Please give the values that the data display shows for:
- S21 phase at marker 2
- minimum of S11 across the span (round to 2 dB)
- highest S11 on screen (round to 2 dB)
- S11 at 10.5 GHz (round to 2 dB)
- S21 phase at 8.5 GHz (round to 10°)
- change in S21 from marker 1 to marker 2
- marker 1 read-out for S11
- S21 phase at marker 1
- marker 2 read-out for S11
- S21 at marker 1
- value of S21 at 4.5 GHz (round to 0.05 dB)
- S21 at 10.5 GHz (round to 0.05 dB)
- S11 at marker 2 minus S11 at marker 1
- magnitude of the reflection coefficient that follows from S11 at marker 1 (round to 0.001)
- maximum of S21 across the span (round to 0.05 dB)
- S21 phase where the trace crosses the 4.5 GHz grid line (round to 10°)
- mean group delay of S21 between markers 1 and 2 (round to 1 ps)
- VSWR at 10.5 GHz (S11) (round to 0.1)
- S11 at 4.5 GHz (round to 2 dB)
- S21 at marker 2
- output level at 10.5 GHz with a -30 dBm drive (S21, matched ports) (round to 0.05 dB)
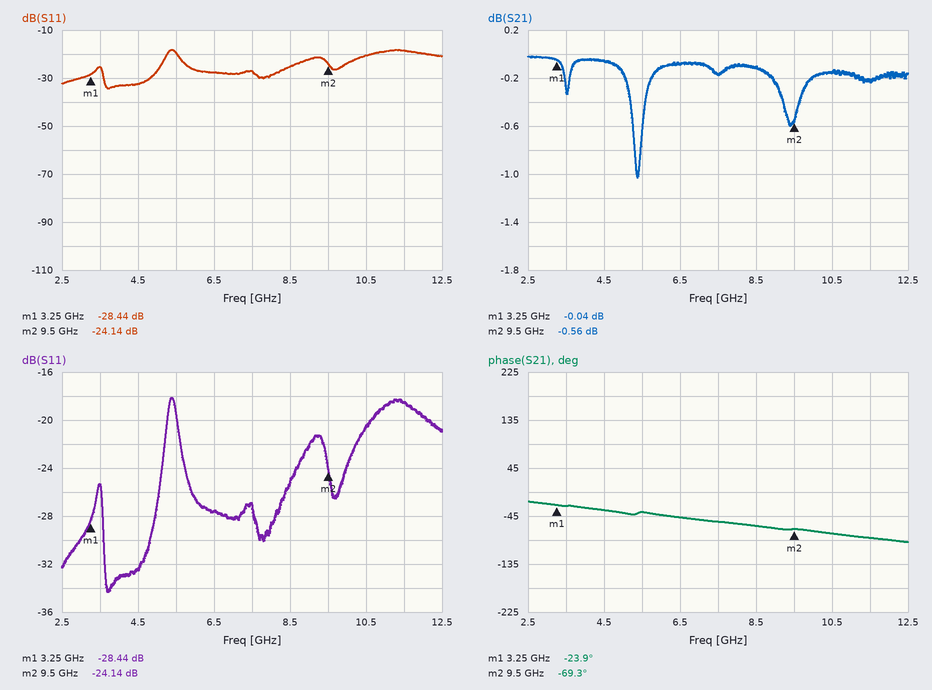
-69.3°
-34 dB
-18 dB
-20 dB
-60°
-0.52 dB
-28.44 dB
-23.9°
-24.14 dB
-0.04 dB
-0.05 dB
-0.15 dB
4.30 dB
0.038
0.00 dB
-30°
20 ps
1.2
-32 dB
-0.56 dB
-30.15 dBm
